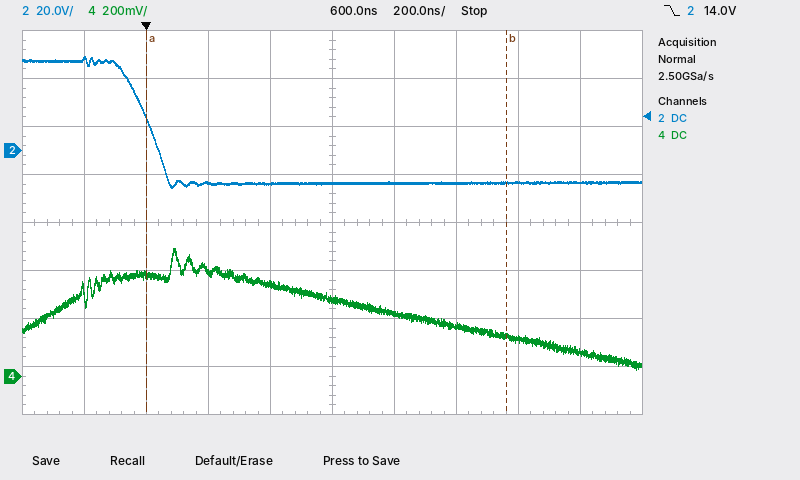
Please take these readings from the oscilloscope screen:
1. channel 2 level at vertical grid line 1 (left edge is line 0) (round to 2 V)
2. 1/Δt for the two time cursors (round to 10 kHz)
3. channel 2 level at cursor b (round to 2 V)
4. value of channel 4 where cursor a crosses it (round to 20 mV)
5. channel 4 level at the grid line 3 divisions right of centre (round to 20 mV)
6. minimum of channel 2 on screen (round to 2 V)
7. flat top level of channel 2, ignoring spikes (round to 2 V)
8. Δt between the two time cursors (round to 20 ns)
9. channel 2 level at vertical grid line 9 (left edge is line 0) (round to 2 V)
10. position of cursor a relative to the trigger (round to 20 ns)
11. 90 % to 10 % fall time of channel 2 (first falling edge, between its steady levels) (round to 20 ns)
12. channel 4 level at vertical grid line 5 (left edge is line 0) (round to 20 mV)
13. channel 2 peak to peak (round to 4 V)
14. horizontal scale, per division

38 V
860 kHz
-14 V
420 mV
160 mV
-16 V
38 V
1.16 µs
-14 V
0 ns
140 ns
320 mV
56 V
200 ns
